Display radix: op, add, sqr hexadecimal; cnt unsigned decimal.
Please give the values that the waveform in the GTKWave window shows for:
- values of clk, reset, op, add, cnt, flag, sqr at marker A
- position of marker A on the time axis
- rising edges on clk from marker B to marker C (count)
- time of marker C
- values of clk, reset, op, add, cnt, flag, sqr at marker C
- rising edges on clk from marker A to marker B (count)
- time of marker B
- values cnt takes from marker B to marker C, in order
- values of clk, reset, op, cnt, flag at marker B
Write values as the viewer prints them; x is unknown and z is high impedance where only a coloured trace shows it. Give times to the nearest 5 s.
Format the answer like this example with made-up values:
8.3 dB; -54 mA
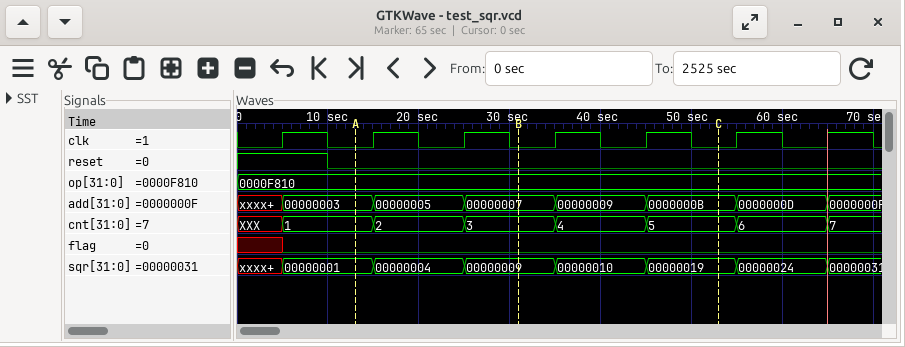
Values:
clk=0, reset=0, op=0000F810, add=00000003, cnt=1, flag=0, sqr=00000001; 15 s; 2; 55 s; clk=0, reset=0, op=0000F810, add=0000000B, cnt=5, flag=0, sqr=00000019; 2; 30 s; 3, 4, 5; clk=0, reset=0, op=0000F810, cnt=3, flag=0
